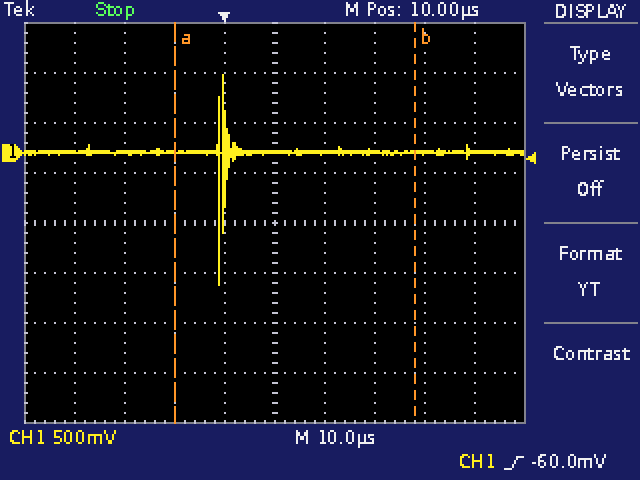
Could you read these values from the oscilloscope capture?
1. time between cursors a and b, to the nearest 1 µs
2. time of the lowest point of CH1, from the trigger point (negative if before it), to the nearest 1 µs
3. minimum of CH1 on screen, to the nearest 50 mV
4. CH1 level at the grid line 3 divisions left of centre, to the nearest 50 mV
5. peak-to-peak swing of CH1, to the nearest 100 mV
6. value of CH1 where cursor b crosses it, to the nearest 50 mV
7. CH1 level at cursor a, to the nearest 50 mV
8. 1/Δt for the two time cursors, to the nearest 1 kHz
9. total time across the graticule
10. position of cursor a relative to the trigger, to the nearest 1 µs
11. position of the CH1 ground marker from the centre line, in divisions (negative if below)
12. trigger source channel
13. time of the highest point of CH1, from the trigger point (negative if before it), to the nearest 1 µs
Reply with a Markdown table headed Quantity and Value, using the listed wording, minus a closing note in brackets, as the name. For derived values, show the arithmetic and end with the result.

| Quantity | Value |
|---|---|
| time between cursors a and b, to the nearest 1 µs | 48 µs |
| time of the lowest point of CH1, from the trigger point (negative if before it), to the nearest 1 µs | -1 µs |
| minimum of CH1 on screen, to the nearest 50 mV | -1.30 V |
| CH1 level at the grid line 3 divisions left of centre, to the nearest 50 mV | 0 mV |
| peak-to-peak swing of CH1, to the nearest 100 mV | 2.10 V |
| value of CH1 where cursor b crosses it, to the nearest 50 mV | 0 mV |
| CH1 level at cursor a, to the nearest 50 mV | 0 mV |
| 1/Δt for the two time cursors, to the nearest 1 kHz | 1 / 48 µs ≈ 21 kHz |
| total time across the graticule | 100 µs |
| position of cursor a relative to the trigger, to the nearest 1 µs | -10 µs |
| position of the CH1 ground marker from the centre line, in divisions | +1.4 div |
| trigger source channel | CH1 |
| time of the highest point of CH1, from the trigger point (negative if before it), to the nearest 1 µs | 0 µs |
